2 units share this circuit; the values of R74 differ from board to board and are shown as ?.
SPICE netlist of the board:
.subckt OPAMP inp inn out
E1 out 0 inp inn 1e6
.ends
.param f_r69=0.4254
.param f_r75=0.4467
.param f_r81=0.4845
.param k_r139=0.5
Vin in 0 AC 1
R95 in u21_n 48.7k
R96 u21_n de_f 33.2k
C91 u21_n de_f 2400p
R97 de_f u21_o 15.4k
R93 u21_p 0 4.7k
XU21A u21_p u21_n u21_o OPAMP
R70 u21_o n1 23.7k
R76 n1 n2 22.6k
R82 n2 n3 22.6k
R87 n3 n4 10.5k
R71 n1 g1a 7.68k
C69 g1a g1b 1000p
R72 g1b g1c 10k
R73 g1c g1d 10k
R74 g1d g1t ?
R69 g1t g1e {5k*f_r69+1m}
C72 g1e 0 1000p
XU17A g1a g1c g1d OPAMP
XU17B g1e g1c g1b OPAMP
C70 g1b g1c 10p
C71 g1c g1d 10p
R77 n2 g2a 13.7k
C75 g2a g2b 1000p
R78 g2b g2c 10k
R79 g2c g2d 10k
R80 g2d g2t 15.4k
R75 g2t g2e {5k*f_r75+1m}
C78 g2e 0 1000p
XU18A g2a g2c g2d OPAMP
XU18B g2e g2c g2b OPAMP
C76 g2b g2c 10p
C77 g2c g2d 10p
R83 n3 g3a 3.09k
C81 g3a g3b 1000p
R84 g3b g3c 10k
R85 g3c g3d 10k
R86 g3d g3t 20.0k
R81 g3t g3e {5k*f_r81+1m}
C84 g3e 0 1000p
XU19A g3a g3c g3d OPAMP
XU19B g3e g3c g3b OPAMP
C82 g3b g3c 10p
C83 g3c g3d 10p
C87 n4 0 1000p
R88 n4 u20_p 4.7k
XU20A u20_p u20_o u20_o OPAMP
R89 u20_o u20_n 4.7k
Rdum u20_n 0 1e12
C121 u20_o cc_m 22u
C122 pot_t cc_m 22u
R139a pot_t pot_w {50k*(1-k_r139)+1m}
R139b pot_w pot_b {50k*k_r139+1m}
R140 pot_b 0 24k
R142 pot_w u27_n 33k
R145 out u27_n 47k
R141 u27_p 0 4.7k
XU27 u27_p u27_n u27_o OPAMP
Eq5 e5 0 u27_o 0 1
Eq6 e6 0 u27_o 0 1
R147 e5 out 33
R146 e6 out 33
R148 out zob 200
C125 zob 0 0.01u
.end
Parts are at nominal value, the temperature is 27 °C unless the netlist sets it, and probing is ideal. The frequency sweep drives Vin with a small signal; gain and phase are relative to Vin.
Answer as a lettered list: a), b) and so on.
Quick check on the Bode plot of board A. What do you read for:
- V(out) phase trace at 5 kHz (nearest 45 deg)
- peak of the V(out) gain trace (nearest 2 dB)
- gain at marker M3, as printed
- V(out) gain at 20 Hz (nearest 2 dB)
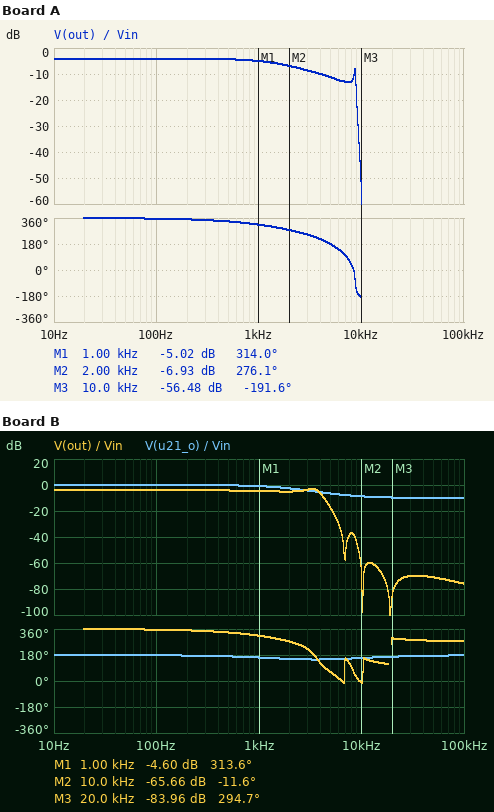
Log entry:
a) 180 deg
b) -4 dB
c) -56.48 dB
d) -4 dB
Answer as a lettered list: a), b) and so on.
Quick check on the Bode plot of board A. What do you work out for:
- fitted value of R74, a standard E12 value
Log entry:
a) 18 kΩ
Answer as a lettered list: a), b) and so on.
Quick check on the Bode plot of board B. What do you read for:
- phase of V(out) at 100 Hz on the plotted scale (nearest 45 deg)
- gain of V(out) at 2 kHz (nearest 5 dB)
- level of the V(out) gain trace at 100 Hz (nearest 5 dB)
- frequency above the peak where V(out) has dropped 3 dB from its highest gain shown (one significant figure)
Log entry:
a) 360 deg
b) -5 dB
c) -5 dB
d) 4 kHz
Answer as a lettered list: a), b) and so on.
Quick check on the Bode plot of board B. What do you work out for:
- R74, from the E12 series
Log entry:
a) 68 kΩ
